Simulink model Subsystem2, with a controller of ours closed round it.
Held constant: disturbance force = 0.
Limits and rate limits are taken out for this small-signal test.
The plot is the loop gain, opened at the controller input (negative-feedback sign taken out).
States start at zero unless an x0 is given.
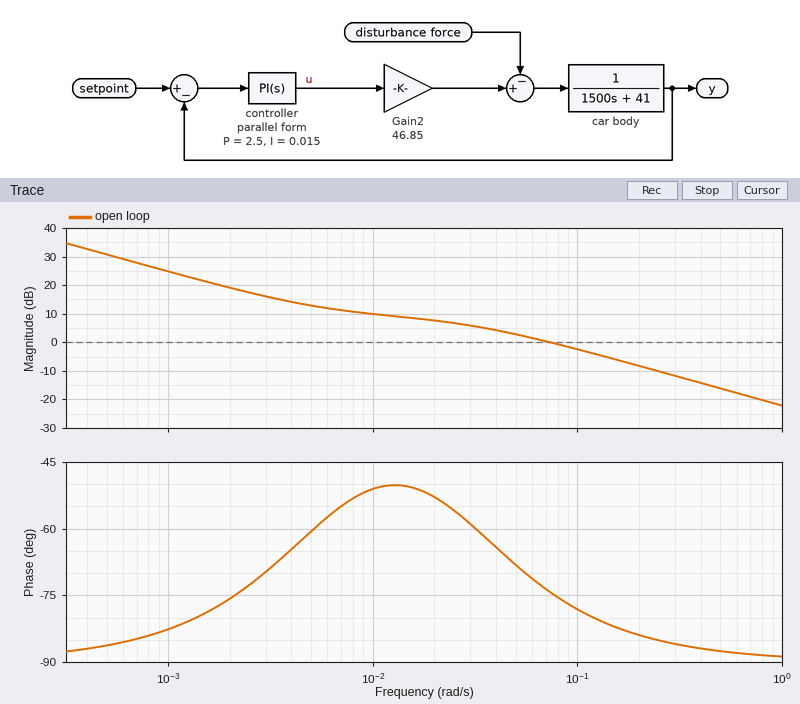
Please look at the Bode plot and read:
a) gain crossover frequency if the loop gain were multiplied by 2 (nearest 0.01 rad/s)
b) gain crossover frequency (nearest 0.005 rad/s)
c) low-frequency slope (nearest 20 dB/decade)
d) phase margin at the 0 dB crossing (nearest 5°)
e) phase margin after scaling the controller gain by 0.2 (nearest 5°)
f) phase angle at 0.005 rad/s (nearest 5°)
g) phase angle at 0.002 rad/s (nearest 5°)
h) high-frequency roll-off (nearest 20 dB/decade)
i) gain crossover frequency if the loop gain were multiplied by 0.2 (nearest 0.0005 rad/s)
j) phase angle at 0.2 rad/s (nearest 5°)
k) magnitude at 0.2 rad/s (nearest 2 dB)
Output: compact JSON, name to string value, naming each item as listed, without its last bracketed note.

{"gain crossover frequency if the loop gain were multiplied by 2": "0.15 rad/s", "gain crossover frequency": "0.075 rad/s", "low-frequency slope": "-20 dB/decade", "phase margin at the 0 dB crossing": "105°", "phase margin after scaling the controller gain by 0.2": "115°", "phase angle at 0.005 rad/s": "-60°", "phase angle at 0.002 rad/s": "-75°", "high-frequency roll-off": "-20 dB/decade", "gain crossover frequency if the loop gain were multiplied by 0.2": "0.0040 rad/s", "phase angle at 0.2 rad/s": "-85°", "magnitude at 0.2 rad/s": "-8 dB"}
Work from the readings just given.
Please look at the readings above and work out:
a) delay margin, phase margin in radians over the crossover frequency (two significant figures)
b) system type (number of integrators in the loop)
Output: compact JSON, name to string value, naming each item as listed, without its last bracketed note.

{"delay margin, phase margin in radians over the crossover frequency": "24 s", "system type": "1"}
